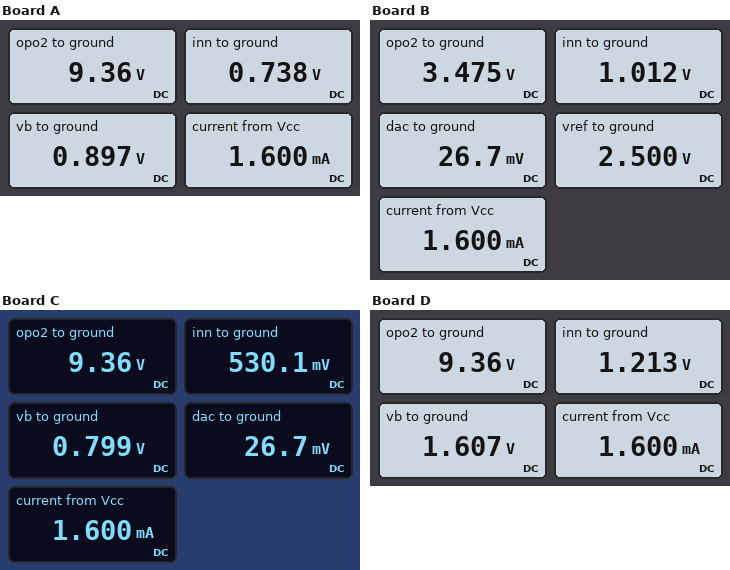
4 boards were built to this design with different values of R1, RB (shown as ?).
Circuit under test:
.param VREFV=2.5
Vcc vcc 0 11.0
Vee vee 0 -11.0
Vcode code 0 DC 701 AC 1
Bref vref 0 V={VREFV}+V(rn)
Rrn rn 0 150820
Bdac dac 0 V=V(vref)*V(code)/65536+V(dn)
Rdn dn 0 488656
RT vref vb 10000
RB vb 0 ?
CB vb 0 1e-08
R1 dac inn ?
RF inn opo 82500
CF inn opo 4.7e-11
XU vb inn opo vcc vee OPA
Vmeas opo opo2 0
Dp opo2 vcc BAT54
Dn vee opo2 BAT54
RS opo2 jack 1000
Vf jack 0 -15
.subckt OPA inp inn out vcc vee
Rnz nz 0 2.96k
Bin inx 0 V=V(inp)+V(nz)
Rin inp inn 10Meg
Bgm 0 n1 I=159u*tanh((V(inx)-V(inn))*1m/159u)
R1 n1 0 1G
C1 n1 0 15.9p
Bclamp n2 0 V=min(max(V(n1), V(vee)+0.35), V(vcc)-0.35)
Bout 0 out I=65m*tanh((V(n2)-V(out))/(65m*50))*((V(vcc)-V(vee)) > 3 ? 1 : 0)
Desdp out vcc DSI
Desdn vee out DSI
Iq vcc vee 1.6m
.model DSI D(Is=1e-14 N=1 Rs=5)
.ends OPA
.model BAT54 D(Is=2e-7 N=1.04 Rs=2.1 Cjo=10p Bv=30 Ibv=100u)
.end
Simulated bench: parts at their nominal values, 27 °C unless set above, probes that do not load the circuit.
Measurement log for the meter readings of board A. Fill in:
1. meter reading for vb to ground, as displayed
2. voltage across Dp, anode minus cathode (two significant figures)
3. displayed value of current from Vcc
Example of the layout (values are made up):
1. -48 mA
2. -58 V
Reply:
1. 0.897 V
2. -1.6 V
3. 1.600 mA
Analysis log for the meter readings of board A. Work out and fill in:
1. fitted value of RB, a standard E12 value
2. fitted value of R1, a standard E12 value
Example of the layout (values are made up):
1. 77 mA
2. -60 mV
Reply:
1. 5.6 kΩ
2. 6.8 kΩ
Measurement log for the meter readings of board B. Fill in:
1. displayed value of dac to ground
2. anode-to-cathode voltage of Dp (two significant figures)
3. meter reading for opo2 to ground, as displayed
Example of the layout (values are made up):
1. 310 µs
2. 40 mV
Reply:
1. 26.7 mV
2. -7.5 V
3. 3.475 V
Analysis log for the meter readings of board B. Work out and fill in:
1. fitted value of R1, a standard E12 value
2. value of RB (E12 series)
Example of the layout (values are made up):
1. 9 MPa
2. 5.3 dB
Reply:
1. 33 kΩ
2. 6.8 kΩ
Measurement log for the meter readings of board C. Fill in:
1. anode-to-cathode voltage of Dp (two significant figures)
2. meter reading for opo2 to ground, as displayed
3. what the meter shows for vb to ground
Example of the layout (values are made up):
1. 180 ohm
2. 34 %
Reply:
1. -1.6 V
2. 9.36 V
3. 0.799 V
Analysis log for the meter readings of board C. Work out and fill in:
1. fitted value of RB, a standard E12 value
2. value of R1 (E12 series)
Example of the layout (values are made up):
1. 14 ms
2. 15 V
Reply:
1. 4.7 kΩ
2. 4.7 kΩ
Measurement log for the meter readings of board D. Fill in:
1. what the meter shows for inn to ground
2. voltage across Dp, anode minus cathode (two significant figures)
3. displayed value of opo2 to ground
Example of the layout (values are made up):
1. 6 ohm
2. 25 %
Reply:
1. 1.213 V
2. -1.6 V
3. 9.36 V
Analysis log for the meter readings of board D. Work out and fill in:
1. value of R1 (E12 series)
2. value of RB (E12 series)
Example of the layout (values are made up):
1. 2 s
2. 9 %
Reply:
1. 12 kΩ
2. 18 kΩ
